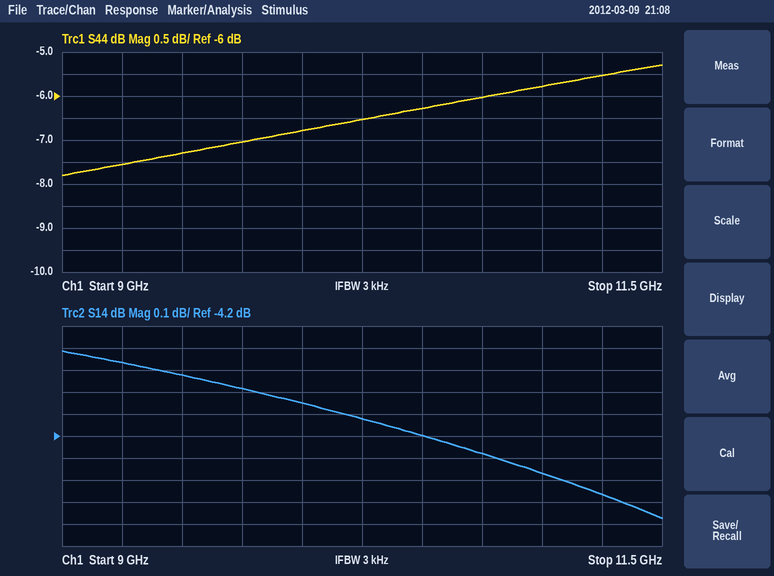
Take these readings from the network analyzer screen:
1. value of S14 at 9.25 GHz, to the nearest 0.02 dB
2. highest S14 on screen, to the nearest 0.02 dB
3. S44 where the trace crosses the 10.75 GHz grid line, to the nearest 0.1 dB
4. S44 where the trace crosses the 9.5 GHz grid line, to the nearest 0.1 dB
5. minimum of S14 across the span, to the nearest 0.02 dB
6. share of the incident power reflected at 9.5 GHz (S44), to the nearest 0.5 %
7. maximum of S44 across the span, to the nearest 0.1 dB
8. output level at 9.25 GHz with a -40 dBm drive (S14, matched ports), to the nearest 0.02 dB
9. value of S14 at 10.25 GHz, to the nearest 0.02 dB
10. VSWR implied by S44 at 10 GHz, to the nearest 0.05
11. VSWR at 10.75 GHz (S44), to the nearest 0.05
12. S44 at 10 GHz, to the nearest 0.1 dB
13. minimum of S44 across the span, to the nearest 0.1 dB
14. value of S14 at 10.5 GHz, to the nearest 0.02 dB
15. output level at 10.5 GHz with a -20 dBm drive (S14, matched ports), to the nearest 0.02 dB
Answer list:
-3.86 dB
-3.82 dB
-6.0 dB
-7.3 dB
-4.58 dB
18.5 %
-5.3 dB
-43.86 dBm
-4.12 dB
2.70
3.00
-6.8 dB
-7.8 dB
-4.20 dB
-24.20 dBm
